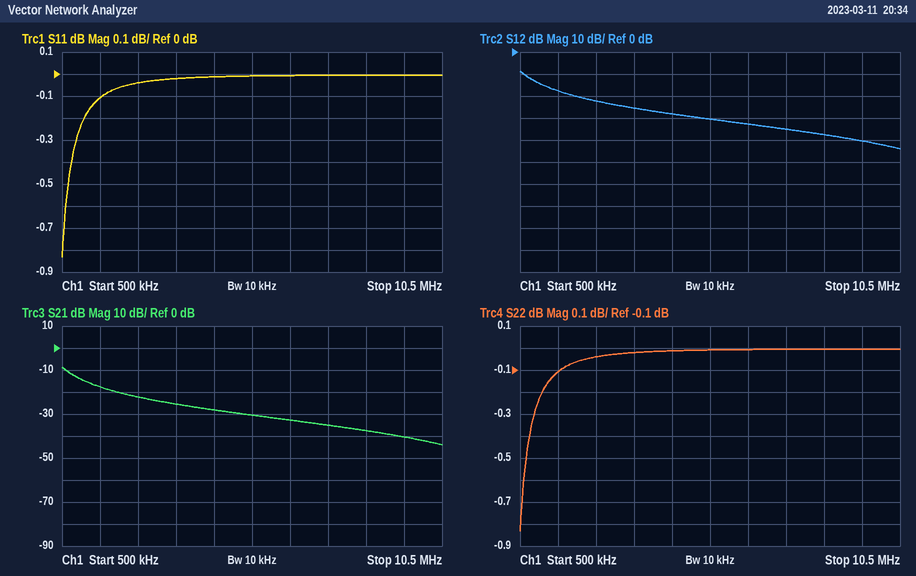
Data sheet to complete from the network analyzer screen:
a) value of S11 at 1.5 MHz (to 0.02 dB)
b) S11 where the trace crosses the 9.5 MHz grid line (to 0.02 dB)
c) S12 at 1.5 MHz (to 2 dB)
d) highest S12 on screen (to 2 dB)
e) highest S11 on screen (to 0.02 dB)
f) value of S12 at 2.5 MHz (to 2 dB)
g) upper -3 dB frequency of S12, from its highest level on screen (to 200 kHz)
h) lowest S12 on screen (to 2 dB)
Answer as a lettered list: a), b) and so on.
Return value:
a) -0.10 dB
b) 0.00 dB
c) -18 dB
d) -8 dB
e) 0.00 dB
f) -22 dB
g) 800 kHz
h) -44 dB
